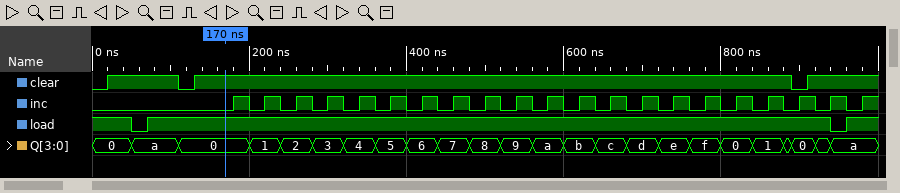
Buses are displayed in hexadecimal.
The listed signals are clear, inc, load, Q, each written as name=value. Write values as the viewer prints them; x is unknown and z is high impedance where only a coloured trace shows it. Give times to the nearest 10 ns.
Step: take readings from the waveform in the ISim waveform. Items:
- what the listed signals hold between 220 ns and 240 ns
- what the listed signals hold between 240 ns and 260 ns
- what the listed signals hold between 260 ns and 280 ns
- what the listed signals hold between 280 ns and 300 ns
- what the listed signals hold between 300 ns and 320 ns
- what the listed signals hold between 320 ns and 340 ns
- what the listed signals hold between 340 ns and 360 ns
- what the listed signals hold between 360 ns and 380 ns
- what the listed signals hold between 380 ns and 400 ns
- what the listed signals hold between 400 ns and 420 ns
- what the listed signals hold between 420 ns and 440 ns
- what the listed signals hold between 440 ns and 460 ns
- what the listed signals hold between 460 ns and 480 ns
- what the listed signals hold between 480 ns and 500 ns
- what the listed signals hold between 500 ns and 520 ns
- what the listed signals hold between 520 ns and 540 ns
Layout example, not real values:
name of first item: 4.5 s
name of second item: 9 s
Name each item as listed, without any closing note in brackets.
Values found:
what the listed signals hold between 220 ns and 240 ns: clear=1, inc=1, load=1, Q=1
what the listed signals hold between 240 ns and 260 ns: clear=1, inc=0, load=1, Q=2
what the listed signals hold between 260 ns and 280 ns: clear=1, inc=1, load=1, Q=2
what the listed signals hold between 280 ns and 300 ns: clear=1, inc=0, load=1, Q=3
what the listed signals hold between 300 ns and 320 ns: clear=1, inc=1, load=1, Q=3
what the listed signals hold between 320 ns and 340 ns: clear=1, inc=0, load=1, Q=4
what the listed signals hold between 340 ns and 360 ns: clear=1, inc=1, load=1, Q=4
what the listed signals hold between 360 ns and 380 ns: clear=1, inc=0, load=1, Q=5
what the listed signals hold between 380 ns and 400 ns: clear=1, inc=1, load=1, Q=5
what the listed signals hold between 400 ns and 420 ns: clear=1, inc=0, load=1, Q=6
what the listed signals hold between 420 ns and 440 ns: clear=1, inc=1, load=1, Q=6
what the listed signals hold between 440 ns and 460 ns: clear=1, inc=0, load=1, Q=7
what the listed signals hold between 460 ns and 480 ns: clear=1, inc=1, load=1, Q=7
what the listed signals hold between 480 ns and 500 ns: clear=1, inc=0, load=1, Q=8
what the listed signals hold between 500 ns and 520 ns: clear=1, inc=1, load=1, Q=8
what the listed signals hold between 520 ns and 540 ns: clear=1, inc=0, load=1, Q=9
